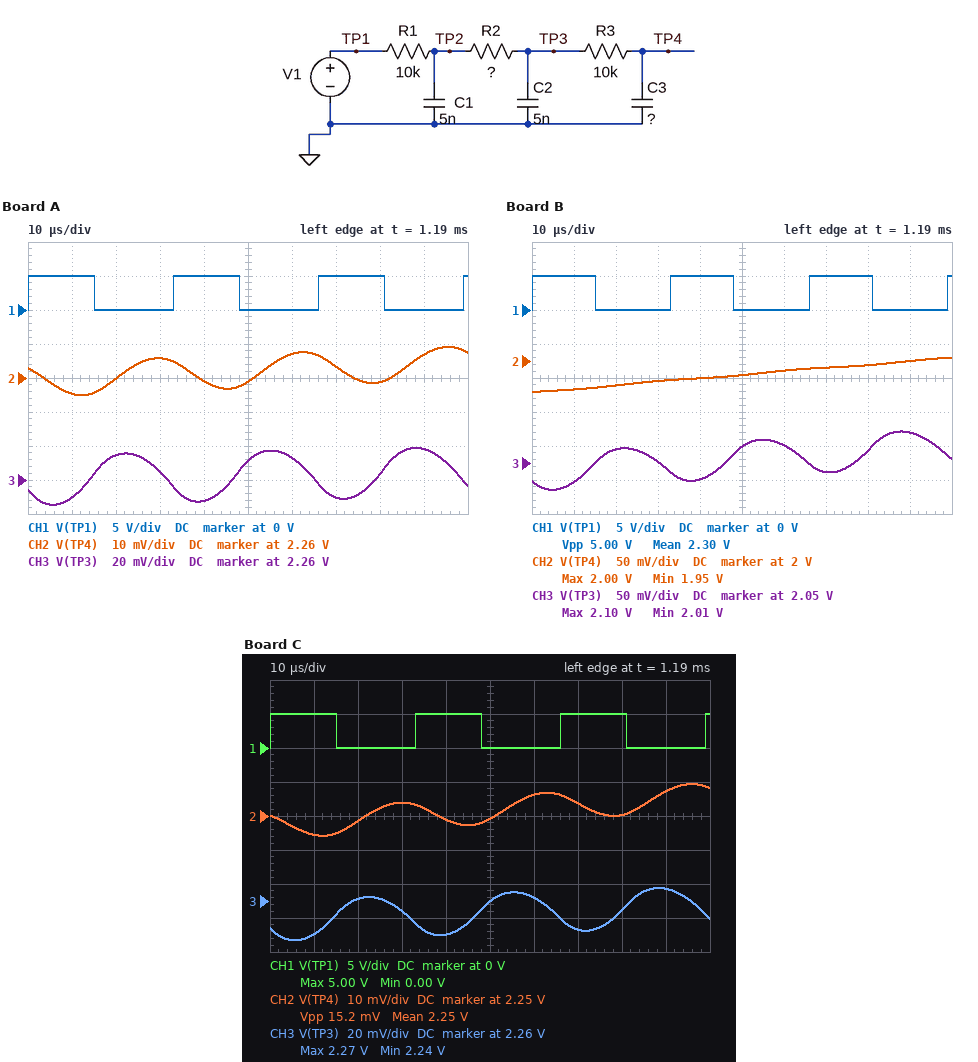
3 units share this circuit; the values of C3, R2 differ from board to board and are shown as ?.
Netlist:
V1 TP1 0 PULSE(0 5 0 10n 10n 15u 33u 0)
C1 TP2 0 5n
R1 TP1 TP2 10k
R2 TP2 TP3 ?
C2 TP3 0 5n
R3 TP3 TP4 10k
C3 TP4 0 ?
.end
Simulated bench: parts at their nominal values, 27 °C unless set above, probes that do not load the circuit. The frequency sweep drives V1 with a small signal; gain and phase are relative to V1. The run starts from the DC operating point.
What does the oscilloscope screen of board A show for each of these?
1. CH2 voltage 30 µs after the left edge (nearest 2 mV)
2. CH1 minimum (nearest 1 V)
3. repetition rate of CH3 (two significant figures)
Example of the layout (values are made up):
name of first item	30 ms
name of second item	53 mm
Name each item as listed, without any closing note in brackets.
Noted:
CH2 voltage 30 µs after the left edge	2.266 V
CH1 minimum	0 V
repetition rate of CH3	31 kHz
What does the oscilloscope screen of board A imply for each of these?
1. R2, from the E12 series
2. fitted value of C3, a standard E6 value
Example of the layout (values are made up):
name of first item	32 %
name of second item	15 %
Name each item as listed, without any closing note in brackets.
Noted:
R2, from the E12 series	22 kΩ
fitted value of C3, a standard E6 value	1.5 nF
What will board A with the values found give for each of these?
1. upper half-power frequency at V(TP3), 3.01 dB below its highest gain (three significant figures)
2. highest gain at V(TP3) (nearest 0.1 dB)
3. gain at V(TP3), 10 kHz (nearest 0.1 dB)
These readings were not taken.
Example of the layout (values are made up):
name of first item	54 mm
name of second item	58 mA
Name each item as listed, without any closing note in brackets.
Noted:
upper half-power frequency at V(TP3), 3.01 dB below its highest gain	681 Hz
highest gain at V(TP3)	0 dB
gain at V(TP3), 10 kHz	-29.2 dB
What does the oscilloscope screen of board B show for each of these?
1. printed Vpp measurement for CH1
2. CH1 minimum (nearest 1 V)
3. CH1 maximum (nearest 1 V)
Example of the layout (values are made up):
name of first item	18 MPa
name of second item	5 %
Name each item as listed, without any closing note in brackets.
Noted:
printed Vpp measurement for CH1	5.00 V
CH1 minimum	0 V
CH1 maximum	5 V
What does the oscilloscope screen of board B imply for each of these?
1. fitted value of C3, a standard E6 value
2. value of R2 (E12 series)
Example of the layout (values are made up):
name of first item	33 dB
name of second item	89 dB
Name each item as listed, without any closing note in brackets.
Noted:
fitted value of C3, a standard E6 value	15 nF
value of R2	12 kΩ
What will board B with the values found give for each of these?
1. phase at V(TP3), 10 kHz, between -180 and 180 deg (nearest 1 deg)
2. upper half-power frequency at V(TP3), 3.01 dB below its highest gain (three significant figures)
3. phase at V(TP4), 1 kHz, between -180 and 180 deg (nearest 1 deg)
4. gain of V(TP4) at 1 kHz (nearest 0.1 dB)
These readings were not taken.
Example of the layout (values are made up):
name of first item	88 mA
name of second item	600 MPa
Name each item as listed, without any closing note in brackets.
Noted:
phase at V(TP3), 10 kHz, between -180 and 180 deg	-123 deg
upper half-power frequency at V(TP3), 3.01 dB below its highest gain	293 Hz
phase at V(TP4), 1 kHz, between -180 and 180 deg	-96 deg
gain of V(TP4) at 1 kHz	-11.9 dB
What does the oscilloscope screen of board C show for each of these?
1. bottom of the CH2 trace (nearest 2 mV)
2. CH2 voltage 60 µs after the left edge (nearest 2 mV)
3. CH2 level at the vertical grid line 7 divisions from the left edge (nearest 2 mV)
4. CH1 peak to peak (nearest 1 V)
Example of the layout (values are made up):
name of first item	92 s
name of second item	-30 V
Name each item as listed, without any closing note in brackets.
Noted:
bottom of the CH2 trace	2.244 V
CH2 voltage 60 µs after the left edge	2.256 V
CH2 level at the vertical grid line 7 divisions from the left edge	2.254 V
CH1 peak to peak	5 V
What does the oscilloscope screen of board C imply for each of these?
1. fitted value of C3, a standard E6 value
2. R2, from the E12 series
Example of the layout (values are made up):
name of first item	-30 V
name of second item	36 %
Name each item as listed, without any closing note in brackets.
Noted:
fitted value of C3, a standard E6 value	1.5 nF
R2, from the E12 series	27 kΩ
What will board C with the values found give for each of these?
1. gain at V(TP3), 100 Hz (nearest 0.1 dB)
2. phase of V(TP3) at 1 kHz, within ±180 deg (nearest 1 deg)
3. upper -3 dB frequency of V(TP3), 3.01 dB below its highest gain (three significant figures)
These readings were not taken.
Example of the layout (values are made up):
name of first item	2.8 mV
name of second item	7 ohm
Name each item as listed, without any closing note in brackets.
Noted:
gain at V(TP3), 100 Hz	-0.1 dB
phase of V(TP3) at 1 kHz, within ±180 deg	-69 deg
upper -3 dB frequency of V(TP3), 3.01 dB below its highest gain	603 Hz
